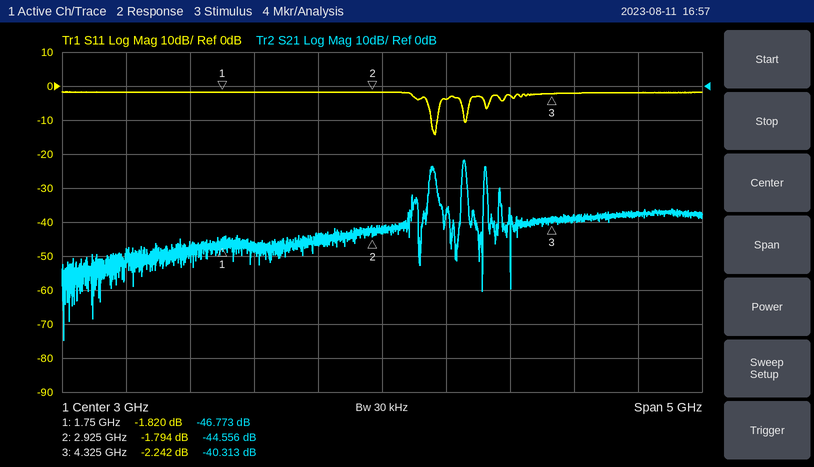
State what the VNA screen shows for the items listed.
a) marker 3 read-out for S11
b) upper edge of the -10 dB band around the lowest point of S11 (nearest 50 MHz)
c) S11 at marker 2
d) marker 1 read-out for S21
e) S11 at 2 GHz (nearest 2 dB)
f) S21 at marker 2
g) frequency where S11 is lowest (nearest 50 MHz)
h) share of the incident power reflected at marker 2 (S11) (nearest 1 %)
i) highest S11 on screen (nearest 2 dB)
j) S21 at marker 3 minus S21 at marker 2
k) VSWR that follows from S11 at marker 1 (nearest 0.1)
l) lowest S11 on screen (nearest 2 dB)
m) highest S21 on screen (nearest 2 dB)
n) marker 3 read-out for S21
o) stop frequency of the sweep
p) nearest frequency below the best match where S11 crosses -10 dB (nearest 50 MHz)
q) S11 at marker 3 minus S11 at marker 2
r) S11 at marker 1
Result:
-2.242 dB
3.45 GHz
-1.794 dB
-46.773 dB
-2 dB
-44.556 dB
3.40 GHz
66 %
-2 dB
4.243 dB
9.6
-14 dB
-22 dB
-40.313 dB
5.5 GHz
3.40 GHz
-0.448 dB
-1.820 dB
